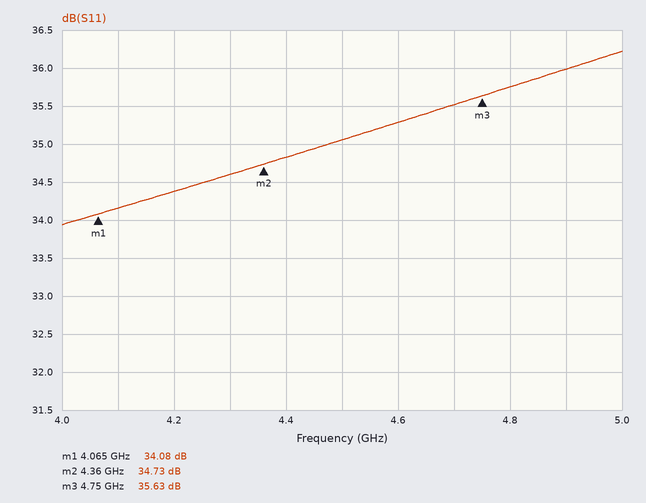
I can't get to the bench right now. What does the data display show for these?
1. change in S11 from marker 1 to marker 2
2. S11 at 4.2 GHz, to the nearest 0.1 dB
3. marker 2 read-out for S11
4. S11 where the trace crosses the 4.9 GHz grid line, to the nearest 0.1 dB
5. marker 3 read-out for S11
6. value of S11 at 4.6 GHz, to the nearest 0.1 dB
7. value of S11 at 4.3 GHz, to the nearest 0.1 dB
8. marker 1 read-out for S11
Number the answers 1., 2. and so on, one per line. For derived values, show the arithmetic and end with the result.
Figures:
1. 34.73 − (34.08) = 0.65 dB
2. 34.4 dB
3. 34.73 dB
4. 36.0 dB
5. 35.63 dB
6. 35.3 dB
7. 34.6 dB
8. 34.08 dB
